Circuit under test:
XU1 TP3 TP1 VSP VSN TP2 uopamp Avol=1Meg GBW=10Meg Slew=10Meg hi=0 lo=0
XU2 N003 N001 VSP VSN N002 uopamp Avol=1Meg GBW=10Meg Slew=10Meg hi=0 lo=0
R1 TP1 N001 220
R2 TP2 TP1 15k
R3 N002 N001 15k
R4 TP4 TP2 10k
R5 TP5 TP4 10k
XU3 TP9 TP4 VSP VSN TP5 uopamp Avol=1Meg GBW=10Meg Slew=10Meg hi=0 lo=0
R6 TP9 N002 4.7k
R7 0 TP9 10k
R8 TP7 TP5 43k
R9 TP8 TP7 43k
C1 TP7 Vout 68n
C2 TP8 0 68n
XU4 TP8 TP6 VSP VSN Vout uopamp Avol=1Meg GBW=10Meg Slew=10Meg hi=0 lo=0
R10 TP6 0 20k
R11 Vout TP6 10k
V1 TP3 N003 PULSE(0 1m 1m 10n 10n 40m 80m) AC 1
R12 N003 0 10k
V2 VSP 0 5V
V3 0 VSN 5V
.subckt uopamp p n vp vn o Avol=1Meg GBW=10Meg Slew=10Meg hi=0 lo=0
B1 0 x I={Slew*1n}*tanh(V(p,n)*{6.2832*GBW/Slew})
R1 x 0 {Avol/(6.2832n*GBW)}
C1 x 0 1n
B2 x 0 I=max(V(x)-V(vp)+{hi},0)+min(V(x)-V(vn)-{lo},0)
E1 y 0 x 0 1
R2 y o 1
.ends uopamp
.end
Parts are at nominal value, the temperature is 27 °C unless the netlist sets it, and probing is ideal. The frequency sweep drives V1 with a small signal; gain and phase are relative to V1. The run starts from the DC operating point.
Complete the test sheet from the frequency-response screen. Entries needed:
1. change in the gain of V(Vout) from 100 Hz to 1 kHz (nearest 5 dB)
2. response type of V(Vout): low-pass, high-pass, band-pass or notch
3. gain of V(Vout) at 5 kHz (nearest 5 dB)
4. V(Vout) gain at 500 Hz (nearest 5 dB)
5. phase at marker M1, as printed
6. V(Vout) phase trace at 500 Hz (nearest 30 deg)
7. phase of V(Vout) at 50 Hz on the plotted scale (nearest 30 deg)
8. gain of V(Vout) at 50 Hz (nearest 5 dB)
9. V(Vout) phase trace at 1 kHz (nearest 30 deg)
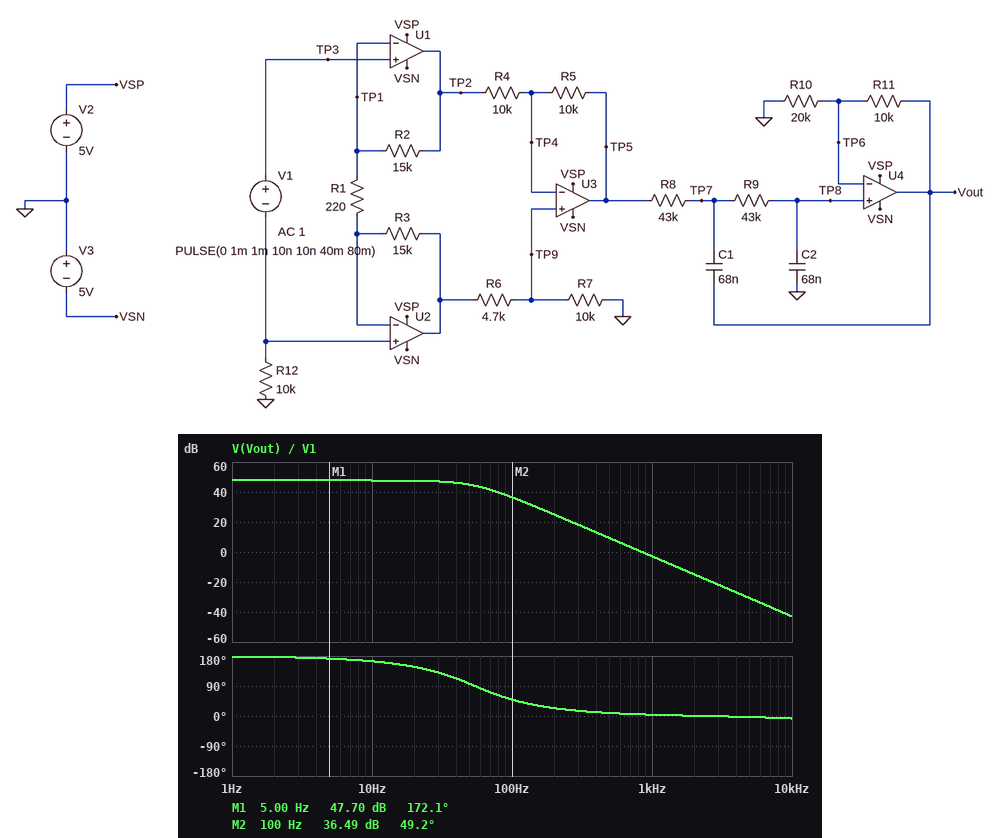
-40 dB
low-pass
-30 dB
10 dB
172.1 deg
0 deg
90 deg
45 dB
0 deg
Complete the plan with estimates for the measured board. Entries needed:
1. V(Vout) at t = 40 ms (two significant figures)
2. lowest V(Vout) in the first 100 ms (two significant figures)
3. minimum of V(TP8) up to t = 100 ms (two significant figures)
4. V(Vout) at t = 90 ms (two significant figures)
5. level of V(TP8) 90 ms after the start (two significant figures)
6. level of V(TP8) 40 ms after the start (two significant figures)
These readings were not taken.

-240 mV
-250 mV
-170 mV
-230 mV
-150 mV
-160 mV
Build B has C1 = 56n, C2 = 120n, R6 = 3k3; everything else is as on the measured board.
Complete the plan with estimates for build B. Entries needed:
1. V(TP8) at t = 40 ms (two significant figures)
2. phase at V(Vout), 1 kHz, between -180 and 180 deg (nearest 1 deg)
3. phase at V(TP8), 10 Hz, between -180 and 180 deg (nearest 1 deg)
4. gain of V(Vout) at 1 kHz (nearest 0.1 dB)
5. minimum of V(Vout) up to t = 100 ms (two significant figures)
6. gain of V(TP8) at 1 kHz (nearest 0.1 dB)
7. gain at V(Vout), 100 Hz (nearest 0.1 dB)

-170 mV
6 deg
149 deg
-5.6 dB
-260 mV
-9.2 dB
31.4 dB
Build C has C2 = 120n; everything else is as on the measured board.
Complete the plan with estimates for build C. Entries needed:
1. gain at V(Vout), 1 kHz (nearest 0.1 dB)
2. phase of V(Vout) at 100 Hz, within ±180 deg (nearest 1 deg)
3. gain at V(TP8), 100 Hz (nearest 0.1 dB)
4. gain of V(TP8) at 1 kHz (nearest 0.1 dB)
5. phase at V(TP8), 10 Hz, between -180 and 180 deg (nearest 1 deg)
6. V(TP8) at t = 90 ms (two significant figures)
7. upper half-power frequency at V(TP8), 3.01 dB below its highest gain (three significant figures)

-7.8 dB
48 deg
26.7 dB
-11.3 dB
149 deg
-100 mV
21.9 Hz
